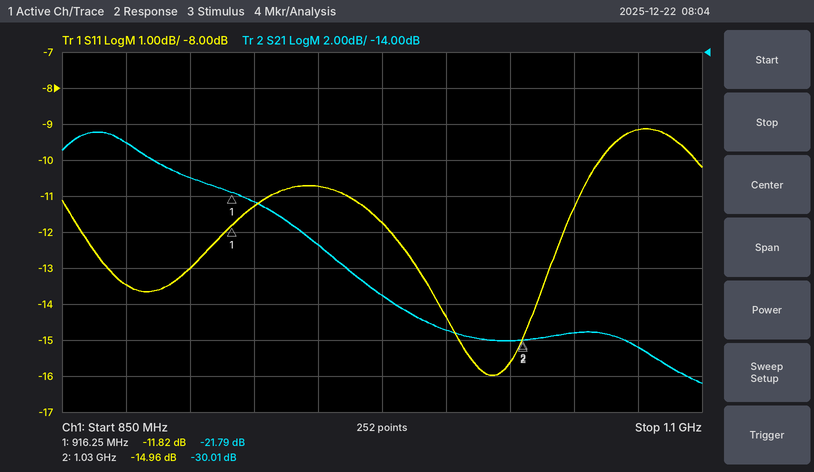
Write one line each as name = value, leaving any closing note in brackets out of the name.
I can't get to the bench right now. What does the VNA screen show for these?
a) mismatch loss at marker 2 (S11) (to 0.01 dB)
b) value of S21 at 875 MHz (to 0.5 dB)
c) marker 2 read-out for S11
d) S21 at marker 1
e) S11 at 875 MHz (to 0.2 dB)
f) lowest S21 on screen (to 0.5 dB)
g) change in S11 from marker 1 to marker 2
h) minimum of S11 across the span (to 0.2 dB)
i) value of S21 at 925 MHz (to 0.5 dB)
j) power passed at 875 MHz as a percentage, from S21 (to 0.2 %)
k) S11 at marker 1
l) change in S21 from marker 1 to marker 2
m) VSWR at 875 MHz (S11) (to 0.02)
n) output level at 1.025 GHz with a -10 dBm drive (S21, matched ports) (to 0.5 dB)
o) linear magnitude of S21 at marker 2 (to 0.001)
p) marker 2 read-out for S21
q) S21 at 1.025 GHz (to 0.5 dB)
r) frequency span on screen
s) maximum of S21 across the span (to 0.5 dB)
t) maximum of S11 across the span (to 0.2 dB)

mismatch loss at marker 2 (S11) = 0.14 dB
value of S21 at 875 MHz = -19.0 dB
marker 2 read-out for S11 = -14.96 dB
S21 at marker 1 = -21.79 dB
S11 at 875 MHz = -13.4 dB
lowest S21 on screen = -32.5 dB
change in S11 from marker 1 to marker 2 = -3.14 dB
minimum of S11 across the span = -16.0 dB
value of S21 at 925 MHz = -22.5 dB
power passed at 875 MHz as a percentage, from S21 = 1.2 %
S11 at marker 1 = -11.82 dB
change in S21 from marker 1 to marker 2 = -8.22 dB
VSWR at 875 MHz (S11) = 1.54
output level at 1.025 GHz with a -10 dBm drive (S21, matched ports) = -40.0 dBm
linear magnitude of S21 at marker 2 = 0.032
marker 2 read-out for S21 = -30.01 dB
S21 at 1.025 GHz = -30.0 dB
frequency span on screen = 250 MHz
maximum of S21 across the span = -18.5 dB
maximum of S11 across the span = -9.2 dB
